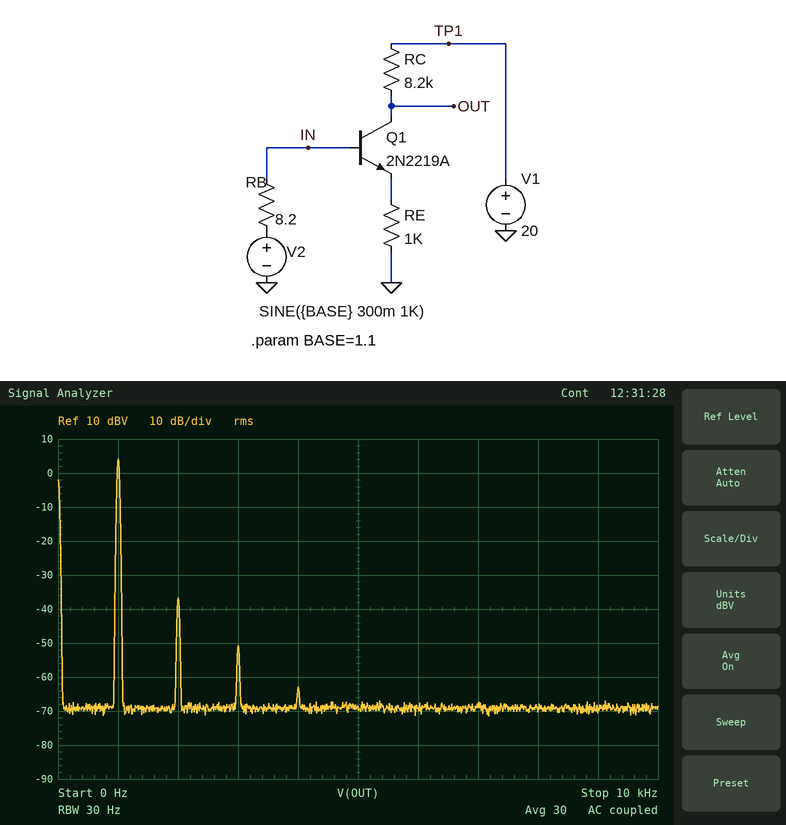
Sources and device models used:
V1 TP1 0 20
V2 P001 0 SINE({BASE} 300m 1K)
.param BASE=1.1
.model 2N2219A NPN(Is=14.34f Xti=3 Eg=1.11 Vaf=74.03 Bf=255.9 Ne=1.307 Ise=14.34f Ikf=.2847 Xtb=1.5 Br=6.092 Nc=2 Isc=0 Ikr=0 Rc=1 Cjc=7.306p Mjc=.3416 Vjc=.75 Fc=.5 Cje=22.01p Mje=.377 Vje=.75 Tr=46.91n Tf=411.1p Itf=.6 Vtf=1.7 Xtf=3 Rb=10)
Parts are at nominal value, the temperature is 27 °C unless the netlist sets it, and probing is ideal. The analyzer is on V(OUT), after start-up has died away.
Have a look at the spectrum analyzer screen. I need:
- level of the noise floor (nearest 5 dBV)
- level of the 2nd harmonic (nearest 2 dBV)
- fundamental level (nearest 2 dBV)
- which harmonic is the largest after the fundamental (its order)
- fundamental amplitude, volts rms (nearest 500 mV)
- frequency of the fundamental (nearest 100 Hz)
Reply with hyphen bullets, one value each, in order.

- -70 dBV
- -36 dBV
- 4 dBV
- 2
- 1.5 V
- 1.0 kHz
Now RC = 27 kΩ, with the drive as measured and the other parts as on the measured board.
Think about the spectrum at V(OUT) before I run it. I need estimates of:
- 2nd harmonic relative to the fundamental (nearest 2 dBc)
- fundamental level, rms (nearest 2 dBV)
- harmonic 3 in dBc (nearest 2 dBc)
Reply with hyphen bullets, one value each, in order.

- -32 dBc
- 14 dBV
- -30 dBc
